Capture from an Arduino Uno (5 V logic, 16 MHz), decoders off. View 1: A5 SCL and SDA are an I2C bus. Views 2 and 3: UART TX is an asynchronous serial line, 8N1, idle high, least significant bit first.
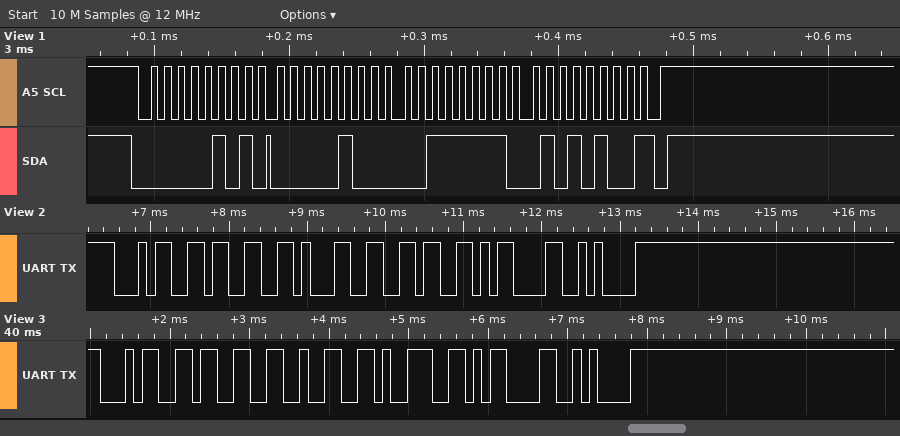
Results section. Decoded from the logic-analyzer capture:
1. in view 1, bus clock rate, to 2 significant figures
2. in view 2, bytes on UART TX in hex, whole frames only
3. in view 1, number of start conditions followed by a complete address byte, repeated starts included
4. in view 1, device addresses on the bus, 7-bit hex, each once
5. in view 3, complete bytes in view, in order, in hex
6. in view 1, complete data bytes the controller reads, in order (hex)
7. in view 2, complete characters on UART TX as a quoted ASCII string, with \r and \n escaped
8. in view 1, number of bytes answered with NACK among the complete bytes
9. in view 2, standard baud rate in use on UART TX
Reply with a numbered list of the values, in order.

1. 100 kHz
2. 34 33 31 36 0D 0A
3. 1
4. 0x02
5. 0x34 0x33 0x32 0x39 0x0D 0x0A
6. 04 3F 54
7. "4316\r\n"
8. 1
9. 9600 baud
